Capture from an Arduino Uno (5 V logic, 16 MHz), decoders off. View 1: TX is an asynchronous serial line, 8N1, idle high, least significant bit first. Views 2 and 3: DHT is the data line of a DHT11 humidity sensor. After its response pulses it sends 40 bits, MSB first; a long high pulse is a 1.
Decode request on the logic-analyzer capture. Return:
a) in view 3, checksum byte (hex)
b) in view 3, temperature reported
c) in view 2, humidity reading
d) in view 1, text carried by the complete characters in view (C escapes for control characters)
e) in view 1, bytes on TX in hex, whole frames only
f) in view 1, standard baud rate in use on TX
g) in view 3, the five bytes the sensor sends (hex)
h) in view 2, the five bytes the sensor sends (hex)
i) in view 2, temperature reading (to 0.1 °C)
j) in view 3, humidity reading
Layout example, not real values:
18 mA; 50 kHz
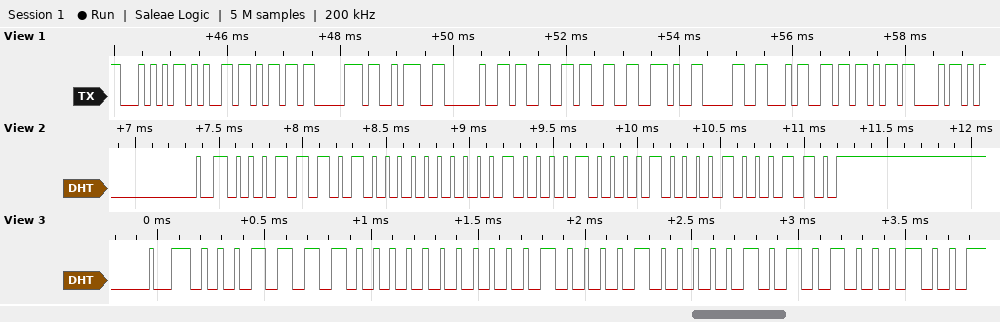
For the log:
0x44; 33.5 °C; 29 %; "Temp: 33.04[C"; 54 65 6D 70 3A 20 33 33 2E 30 34 5B 43; 9600 baud; 1E 00 21 05 44; 1D 00 21 08 46; 33.8 °C; 30 %
